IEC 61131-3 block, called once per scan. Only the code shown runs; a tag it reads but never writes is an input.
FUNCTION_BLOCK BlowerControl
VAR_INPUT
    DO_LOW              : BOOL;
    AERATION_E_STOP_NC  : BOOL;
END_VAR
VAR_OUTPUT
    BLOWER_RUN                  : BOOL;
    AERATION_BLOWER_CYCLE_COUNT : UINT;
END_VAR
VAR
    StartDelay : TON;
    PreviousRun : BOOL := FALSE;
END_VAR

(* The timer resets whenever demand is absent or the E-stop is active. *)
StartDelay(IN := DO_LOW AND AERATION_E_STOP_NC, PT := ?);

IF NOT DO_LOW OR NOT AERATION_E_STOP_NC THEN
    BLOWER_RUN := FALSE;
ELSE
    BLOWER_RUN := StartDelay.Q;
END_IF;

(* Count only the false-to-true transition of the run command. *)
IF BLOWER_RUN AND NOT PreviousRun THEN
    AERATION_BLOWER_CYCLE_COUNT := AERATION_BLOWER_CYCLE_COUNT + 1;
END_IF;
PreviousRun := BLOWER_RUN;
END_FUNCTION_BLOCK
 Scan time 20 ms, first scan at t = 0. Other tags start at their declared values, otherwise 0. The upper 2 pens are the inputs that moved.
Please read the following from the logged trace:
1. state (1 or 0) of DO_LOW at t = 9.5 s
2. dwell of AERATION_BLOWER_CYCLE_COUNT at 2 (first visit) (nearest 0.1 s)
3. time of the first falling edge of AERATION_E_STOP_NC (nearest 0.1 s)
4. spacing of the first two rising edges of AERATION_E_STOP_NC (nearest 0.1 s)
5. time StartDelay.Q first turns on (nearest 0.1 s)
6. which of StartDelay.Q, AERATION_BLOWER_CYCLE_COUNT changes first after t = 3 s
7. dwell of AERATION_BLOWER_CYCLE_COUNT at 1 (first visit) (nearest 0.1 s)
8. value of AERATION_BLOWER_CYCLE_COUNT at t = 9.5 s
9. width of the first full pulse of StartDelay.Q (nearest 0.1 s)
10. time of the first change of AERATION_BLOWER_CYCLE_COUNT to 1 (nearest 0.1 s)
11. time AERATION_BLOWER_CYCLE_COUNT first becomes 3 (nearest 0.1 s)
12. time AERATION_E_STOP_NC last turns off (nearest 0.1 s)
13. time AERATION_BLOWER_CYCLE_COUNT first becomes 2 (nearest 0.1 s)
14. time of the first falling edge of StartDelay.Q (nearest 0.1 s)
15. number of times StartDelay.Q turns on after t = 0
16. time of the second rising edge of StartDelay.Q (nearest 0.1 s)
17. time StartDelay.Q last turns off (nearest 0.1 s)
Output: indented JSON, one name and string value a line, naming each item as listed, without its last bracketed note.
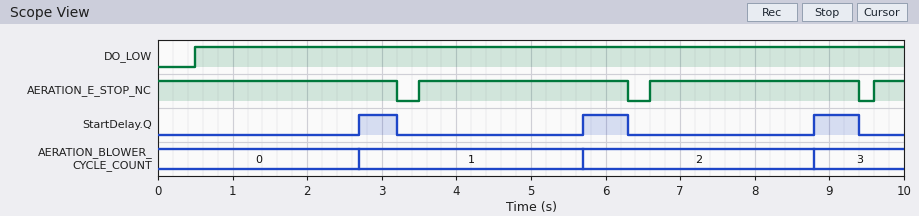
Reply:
{
  "state (1 or 0) of DO_LOW at t = 9.5 s": "1",
  "dwell of AERATION_BLOWER_CYCLE_COUNT at 2 (first visit)": "3.1 s",
  "time of the first falling edge of AERATION_E_STOP_NC": "3.2 s",
  "spacing of the first two rising edges of AERATION_E_STOP_NC": "3.1 s",
  "time StartDelay.Q first turns on": "2.7 s",
  "which of StartDelay.Q, AERATION_BLOWER_CYCLE_COUNT changes first after t = 3 s": "StartDelay.Q",
  "dwell of AERATION_BLOWER_CYCLE_COUNT at 1 (first visit)": "3.0 s",
  "value of AERATION_BLOWER_CYCLE_COUNT at t = 9.5 s": "3",
  "width of the first full pulse of StartDelay.Q": "0.5 s",
  "time of the first change of AERATION_BLOWER_CYCLE_COUNT to 1": "2.7 s",
  "time AERATION_BLOWER_CYCLE_COUNT first becomes 3": "8.8 s",
  "time AERATION_E_STOP_NC last turns off": "9.4 s",
  "time AERATION_BLOWER_CYCLE_COUNT first becomes 2": "5.7 s",
  "time of the first falling edge of StartDelay.Q": "3.2 s",
  "number of times StartDelay.Q turns on after t = 0": "3",
  "time of the second rising edge of StartDelay.Q": "5.7 s",
  "time StartDelay.Q last turns off": "9.4 s"
}
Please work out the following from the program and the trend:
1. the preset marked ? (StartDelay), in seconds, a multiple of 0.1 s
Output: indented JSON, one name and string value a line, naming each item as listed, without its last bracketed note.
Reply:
{
  "the preset marked ? (StartDelay), in seconds, a multiple of 0.1 s": "2.2 s"
}
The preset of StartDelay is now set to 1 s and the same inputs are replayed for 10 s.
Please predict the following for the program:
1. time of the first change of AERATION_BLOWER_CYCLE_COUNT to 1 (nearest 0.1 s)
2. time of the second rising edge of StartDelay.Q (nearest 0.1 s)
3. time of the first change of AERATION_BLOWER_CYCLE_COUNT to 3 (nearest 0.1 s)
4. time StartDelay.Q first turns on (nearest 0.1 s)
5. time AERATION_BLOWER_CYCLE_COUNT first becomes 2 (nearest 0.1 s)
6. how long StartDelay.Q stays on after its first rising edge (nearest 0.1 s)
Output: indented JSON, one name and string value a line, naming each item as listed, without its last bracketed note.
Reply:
{
  "time of the first change of AERATION_BLOWER_CYCLE_COUNT to 1": "1.5 s",
  "time of the second rising edge of StartDelay.Q": "4.5 s",
  "time of the first change of AERATION_BLOWER_CYCLE_COUNT to 3": "7.6 s",
  "time StartDelay.Q first turns on": "1.5 s",
  "time AERATION_BLOWER_CYCLE_COUNT first becomes 2": "4.5 s",
  "how long StartDelay.Q stays on after its first rising edge": "1.7 s"
}
